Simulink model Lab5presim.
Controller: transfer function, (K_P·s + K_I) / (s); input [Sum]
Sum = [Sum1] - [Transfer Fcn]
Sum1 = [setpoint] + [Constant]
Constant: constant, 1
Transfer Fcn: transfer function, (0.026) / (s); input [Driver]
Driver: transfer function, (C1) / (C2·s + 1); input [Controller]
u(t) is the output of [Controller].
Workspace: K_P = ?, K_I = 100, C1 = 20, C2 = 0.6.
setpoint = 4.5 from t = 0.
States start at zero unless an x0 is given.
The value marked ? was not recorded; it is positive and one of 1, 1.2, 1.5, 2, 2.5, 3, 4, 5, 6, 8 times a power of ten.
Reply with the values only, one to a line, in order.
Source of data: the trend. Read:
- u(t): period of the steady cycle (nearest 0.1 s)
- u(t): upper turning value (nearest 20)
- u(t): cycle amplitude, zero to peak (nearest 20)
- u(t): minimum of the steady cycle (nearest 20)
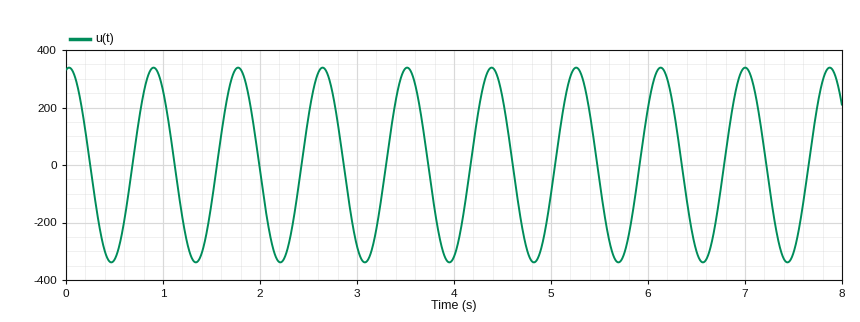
0.9 s
340
340
-340
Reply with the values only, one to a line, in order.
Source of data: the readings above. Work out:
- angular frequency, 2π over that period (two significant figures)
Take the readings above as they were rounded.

7.0 rad/s
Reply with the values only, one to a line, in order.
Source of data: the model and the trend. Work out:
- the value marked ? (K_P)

60
